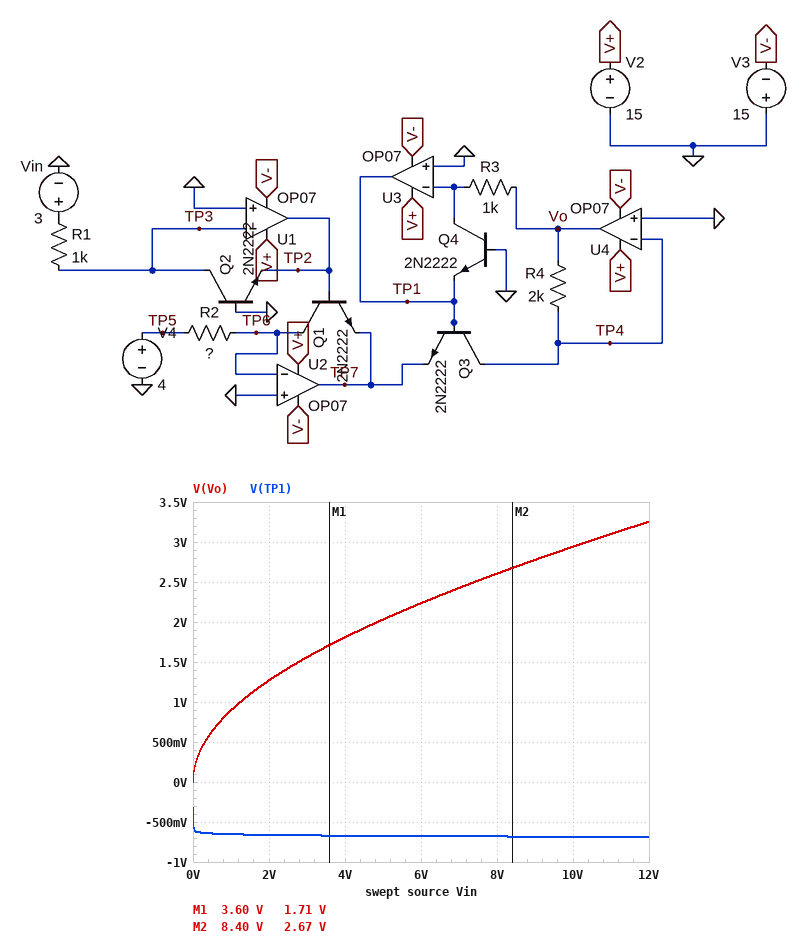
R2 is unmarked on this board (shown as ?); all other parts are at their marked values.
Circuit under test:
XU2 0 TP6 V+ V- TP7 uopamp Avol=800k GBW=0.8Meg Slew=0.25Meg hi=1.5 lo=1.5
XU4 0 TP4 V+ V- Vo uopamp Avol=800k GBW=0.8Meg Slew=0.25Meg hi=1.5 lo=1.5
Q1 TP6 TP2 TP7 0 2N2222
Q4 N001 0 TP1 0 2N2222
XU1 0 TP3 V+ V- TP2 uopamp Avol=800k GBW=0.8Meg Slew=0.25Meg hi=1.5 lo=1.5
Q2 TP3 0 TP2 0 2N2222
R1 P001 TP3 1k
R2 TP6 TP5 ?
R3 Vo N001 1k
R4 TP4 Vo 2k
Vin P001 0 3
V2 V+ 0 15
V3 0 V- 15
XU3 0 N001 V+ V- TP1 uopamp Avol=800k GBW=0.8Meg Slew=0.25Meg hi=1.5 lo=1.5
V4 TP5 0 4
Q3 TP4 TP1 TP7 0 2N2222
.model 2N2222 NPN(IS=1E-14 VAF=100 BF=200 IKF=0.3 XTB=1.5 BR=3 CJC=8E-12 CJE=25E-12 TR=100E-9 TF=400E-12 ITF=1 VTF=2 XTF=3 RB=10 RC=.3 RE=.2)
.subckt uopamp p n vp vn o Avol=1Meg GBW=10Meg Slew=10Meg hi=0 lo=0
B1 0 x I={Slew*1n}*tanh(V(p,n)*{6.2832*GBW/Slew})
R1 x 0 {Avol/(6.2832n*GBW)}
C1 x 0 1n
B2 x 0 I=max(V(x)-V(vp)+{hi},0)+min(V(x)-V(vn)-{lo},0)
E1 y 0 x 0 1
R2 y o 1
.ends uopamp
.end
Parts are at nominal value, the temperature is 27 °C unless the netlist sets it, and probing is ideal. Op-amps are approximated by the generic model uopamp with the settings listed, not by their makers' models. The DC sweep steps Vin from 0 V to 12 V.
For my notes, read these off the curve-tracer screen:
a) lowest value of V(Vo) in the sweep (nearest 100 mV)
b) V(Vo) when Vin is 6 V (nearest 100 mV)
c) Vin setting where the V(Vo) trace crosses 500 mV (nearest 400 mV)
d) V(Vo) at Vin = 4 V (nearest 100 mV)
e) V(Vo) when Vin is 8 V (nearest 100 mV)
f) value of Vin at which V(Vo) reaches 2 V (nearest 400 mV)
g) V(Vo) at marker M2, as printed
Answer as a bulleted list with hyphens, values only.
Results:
- 0 V
- 2.2 V
- 400 mV
- 1.8 V
- 2.6 V
- 4.8 V
- 2.67 V
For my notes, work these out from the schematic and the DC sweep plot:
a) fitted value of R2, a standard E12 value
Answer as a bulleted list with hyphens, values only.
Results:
- 10 kΩ
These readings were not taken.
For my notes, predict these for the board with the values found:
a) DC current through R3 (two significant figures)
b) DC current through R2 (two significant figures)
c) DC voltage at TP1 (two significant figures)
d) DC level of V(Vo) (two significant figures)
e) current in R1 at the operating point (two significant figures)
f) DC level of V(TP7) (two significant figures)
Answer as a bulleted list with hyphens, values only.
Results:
- 1.6 mA
- 400 µA
- -670 mV
- 1.6 V
- 3.0 mA
- -1.3 V
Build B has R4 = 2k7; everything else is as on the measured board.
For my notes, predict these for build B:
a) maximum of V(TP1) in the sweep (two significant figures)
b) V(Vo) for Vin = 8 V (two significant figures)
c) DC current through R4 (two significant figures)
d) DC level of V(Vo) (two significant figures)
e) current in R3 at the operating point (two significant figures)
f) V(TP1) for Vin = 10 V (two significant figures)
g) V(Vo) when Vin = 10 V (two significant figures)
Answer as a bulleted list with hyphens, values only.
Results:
- -330 mV
- 3.0 V
- 670 µA
- 1.8 V
- 1.8 mA
- -690 mV
- 3.4 V
